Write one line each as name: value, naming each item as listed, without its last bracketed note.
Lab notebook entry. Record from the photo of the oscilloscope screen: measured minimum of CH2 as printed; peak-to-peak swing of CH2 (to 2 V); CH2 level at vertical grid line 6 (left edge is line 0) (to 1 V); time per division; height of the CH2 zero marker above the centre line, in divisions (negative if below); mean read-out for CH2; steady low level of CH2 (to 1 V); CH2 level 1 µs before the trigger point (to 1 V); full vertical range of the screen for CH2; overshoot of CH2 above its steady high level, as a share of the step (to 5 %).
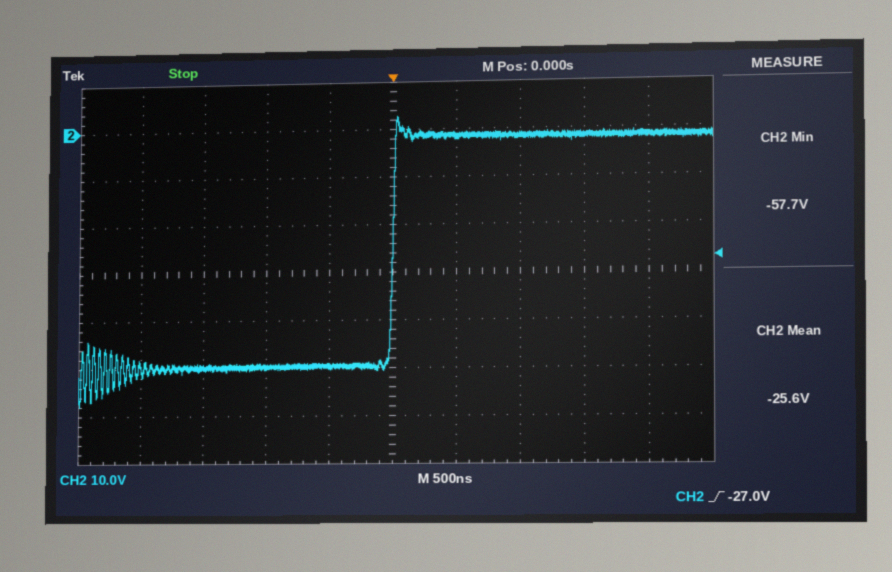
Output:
measured minimum of CH2 as printed: -57.7 V
peak-to-peak swing of CH2: 60 V
CH2 level at vertical grid line 6 (left edge is line 0): -1 V
time per division: 500 ns
height of the CH2 zero marker above the centre line, in divisions: +3.0 div
mean read-out for CH2: -25.6 V
steady low level of CH2: -50 V
CH2 level 1 µs before the trigger point: -50 V
full vertical range of the screen for CH2: 80 V
overshoot of CH2 above its steady high level, as a share of the step: 10 %
